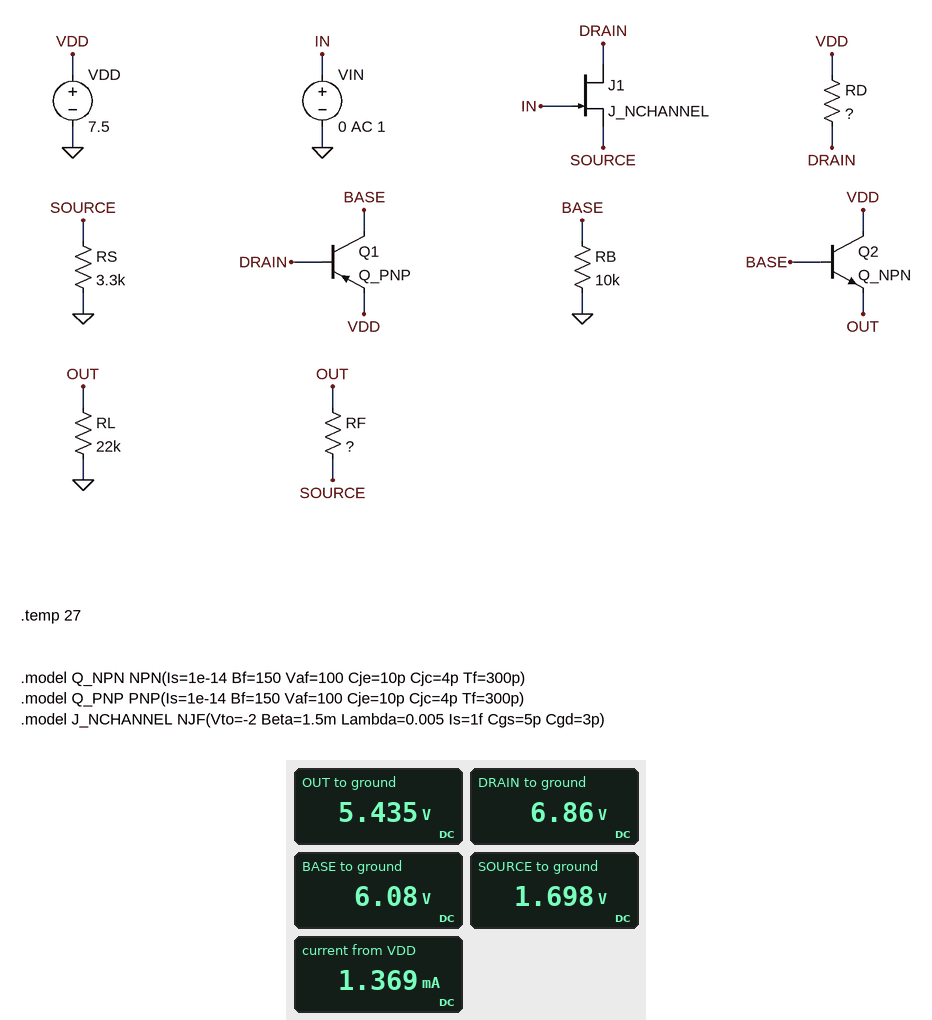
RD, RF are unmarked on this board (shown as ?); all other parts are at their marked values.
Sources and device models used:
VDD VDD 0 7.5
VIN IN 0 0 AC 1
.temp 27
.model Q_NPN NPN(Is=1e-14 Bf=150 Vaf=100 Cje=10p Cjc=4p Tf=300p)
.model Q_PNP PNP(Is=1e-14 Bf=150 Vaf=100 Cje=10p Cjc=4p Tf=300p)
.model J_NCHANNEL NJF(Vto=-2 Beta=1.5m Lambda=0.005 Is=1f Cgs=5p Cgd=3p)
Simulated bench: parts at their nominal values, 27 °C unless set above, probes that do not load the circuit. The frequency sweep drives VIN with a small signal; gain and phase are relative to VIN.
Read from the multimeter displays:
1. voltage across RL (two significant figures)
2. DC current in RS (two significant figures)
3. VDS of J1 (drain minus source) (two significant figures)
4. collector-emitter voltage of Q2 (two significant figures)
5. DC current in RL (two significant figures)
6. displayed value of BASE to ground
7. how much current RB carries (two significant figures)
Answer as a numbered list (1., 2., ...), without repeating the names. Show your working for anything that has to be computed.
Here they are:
1. 5.435 V = 5.4 V
2. (1.698 V) / 3.3 kΩ = 510 µA
3. 6.86 V - 1.698 V = 5.2 V
4. 7.5 V - 5.435 V = 2.1 V
5. (5.435 V) / 22 kΩ = 250 µA
6. 6.08 V
7. (6.08 V) / 10 kΩ = 610 µA
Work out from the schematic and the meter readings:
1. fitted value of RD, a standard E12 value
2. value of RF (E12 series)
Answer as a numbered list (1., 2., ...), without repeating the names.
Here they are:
1. 4.7 kΩ
2. 10 kΩ
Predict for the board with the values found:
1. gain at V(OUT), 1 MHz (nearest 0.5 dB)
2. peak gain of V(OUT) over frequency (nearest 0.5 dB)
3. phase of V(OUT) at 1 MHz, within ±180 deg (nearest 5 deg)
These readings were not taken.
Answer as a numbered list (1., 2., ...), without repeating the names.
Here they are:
1. 11.5 dB
2. 12.0 dB
3. -20 deg
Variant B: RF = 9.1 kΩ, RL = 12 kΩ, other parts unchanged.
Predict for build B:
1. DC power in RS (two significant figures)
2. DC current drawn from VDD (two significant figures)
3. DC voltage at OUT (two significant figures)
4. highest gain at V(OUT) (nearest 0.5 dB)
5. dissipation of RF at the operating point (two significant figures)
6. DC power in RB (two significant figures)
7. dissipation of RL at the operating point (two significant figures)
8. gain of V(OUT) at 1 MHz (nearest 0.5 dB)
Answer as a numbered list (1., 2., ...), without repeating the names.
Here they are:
1. 870 µW
2. 1.5 mA
3. 5.1 V
4. 11.5 dB
5. 1.3 mW
6. 3.3 mW
7. 2.2 mW
8. 11.0 dB
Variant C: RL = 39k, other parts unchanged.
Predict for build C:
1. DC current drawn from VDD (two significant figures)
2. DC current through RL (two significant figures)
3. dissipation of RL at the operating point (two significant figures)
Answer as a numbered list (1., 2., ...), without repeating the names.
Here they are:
1. 1.3 mA
2. 140 µA
3. 760 µW
